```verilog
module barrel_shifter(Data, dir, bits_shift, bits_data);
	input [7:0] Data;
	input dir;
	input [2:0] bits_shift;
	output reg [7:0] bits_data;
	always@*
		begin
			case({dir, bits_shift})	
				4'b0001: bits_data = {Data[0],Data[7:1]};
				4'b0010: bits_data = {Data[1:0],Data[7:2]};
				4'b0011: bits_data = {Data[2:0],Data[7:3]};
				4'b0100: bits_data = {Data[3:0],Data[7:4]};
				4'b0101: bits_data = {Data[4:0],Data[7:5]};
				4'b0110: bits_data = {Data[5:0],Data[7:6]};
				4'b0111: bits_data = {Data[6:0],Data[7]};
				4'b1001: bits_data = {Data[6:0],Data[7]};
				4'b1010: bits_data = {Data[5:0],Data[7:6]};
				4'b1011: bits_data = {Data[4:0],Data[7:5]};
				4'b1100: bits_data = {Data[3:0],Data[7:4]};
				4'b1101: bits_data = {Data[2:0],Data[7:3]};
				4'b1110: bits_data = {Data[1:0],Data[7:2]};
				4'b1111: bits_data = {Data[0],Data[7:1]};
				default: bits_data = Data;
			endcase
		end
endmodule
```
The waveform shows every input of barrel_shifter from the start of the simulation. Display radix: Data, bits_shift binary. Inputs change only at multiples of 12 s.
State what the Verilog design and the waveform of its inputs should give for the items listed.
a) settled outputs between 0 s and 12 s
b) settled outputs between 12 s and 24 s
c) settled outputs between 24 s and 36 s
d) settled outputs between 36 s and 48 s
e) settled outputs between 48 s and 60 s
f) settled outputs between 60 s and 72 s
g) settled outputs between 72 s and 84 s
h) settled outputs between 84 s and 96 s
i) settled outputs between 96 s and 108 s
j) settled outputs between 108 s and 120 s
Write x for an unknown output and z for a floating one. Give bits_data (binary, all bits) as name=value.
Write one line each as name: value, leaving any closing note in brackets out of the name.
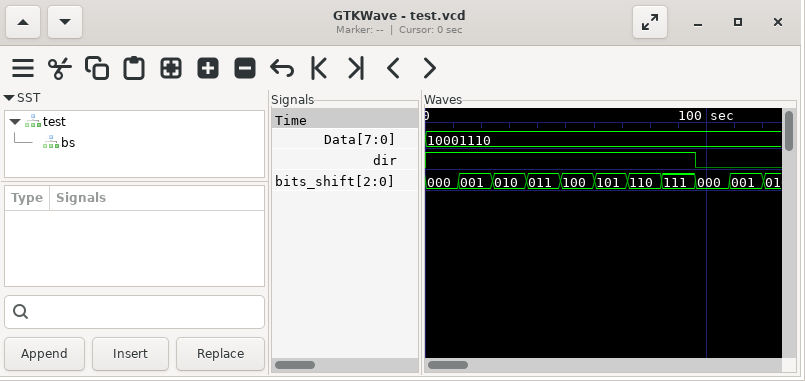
settled outputs between 0 s and 12 s: bits_data=10001110
settled outputs between 12 s and 24 s: bits_data=00011101
settled outputs between 24 s and 36 s: bits_data=00111010
settled outputs between 36 s and 48 s: bits_data=01110100
settled outputs between 48 s and 60 s: bits_data=11101000
settled outputs between 60 s and 72 s: bits_data=11010001
settled outputs between 72 s and 84 s: bits_data=10100011
settled outputs between 84 s and 96 s: bits_data=01000111
settled outputs between 96 s and 108 s: bits_data=10001110
settled outputs between 108 s and 120 s: bits_data=01000111
